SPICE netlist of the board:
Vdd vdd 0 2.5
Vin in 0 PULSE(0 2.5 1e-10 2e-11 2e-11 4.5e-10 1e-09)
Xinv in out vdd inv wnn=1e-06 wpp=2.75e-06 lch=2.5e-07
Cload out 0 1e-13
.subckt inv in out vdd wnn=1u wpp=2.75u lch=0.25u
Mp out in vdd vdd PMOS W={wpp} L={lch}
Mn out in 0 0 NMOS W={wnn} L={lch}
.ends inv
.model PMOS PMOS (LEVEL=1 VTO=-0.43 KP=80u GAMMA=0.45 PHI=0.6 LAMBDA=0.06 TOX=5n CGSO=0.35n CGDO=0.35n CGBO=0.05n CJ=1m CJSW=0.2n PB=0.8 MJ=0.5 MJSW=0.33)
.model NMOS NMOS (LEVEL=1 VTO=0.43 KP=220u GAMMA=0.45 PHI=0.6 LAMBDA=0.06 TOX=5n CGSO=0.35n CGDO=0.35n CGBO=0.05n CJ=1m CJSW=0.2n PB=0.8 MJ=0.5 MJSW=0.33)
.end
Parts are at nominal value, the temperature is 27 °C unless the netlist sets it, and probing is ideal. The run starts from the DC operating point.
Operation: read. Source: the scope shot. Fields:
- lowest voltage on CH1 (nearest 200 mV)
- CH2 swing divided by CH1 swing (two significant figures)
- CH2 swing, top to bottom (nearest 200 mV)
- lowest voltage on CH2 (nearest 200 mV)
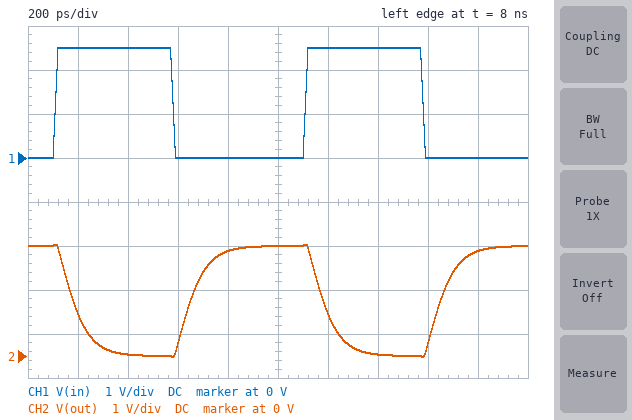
0 V
1.0
2.6 V
0 V
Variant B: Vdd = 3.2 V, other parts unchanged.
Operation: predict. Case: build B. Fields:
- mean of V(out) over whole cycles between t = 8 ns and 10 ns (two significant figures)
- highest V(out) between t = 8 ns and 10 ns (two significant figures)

1.8 V
3.2 V
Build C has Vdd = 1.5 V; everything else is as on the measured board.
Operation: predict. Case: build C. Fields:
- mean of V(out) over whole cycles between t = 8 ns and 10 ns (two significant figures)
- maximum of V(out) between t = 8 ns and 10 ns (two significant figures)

620 mV
1.5 V
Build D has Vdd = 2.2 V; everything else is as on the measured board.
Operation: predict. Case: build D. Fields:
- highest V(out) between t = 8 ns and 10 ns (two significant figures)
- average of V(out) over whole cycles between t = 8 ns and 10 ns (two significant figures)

2.2 V
1.1 V
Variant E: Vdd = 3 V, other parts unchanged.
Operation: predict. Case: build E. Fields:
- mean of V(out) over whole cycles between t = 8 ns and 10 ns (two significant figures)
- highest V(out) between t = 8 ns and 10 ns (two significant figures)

1.7 V
3.0 V
